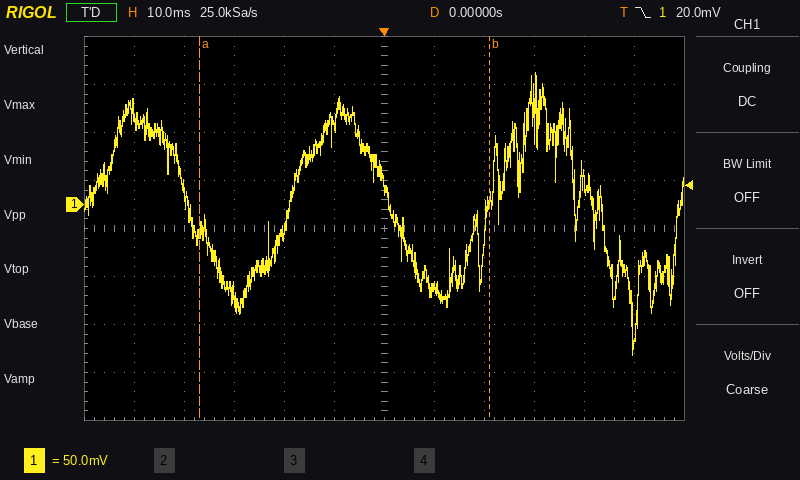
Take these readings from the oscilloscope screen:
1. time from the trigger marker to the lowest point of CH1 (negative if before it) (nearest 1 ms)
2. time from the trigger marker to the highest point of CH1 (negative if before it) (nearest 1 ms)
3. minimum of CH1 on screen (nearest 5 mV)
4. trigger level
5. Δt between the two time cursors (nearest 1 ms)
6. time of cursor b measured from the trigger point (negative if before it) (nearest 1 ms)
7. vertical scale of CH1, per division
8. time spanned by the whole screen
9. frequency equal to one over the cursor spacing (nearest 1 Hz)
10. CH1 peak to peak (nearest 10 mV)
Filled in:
+50 ms
+30 ms
-155 mV
20.0 mV
58 ms
+21 ms
50 mV
120 ms
17 Hz
290 mV
